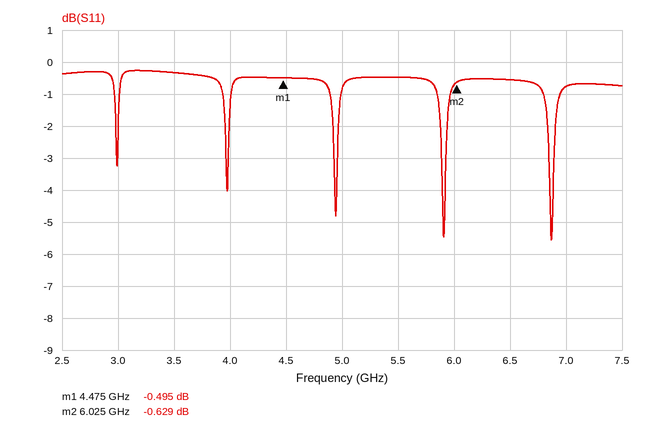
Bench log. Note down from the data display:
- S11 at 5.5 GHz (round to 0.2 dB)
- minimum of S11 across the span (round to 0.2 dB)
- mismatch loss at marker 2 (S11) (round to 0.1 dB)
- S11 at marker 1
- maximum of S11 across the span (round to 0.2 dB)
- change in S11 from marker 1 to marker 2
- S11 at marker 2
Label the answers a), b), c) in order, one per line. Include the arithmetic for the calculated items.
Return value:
a) -0.4 dB
b) -5.6 dB
c) −10 log10(1 − 10^(-0.629/10)) ≈ 8.7 dB
d) -0.495 dB
e) -0.2 dB
f) -0.629 − (-0.495) = -0.134 dB
g) -0.629 dB
